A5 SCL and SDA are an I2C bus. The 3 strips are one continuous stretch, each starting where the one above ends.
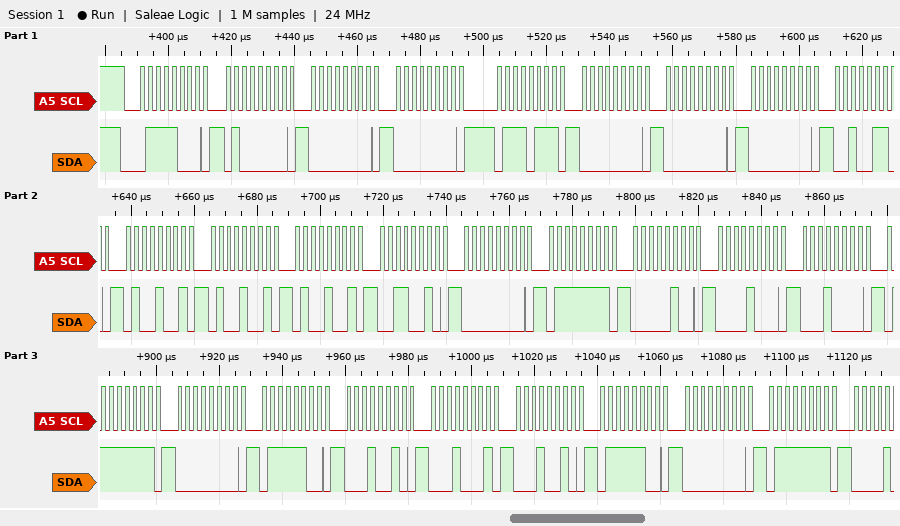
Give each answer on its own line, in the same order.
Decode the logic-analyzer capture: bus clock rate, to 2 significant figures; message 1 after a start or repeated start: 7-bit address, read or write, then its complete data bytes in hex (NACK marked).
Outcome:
400 kHz
0x3C write: 40 00 00 77 00 00 00 26 49 49 49 32 00 7F 04 08 10 7F 00 7C 12 11 12 7C 00 7F
